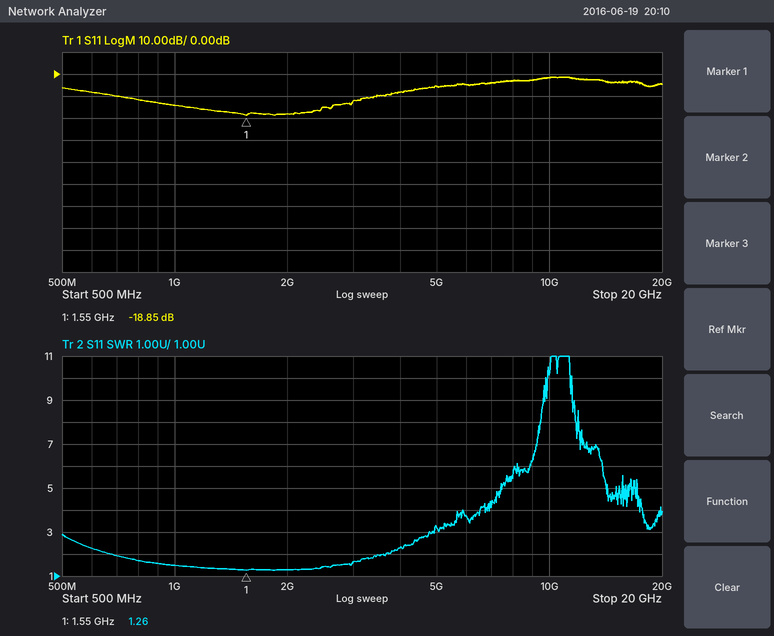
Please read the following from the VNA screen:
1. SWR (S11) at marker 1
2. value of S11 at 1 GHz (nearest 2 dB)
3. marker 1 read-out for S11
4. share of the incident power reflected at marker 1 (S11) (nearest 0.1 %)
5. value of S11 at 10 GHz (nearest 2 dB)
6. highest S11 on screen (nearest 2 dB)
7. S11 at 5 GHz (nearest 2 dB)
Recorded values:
1.26
-14 dB
-18.85 dB
1.3 %
-2 dB
-2 dB
-6 dB
